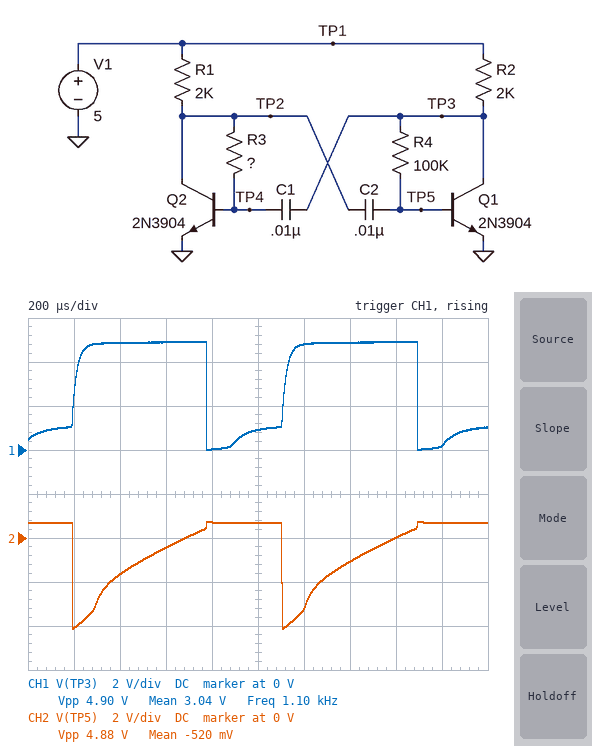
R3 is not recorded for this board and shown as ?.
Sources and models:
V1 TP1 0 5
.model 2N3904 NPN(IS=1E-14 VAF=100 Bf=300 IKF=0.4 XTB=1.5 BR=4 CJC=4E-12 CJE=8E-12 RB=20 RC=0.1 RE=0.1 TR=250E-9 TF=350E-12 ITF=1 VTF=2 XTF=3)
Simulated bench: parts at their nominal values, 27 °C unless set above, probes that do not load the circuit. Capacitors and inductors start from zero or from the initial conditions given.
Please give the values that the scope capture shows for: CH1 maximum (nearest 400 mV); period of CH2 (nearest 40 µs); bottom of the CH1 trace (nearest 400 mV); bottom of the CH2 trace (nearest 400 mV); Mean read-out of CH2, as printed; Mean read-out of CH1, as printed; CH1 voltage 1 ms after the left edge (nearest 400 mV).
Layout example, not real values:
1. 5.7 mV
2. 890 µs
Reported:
1. 4.8 V
2. 920 µs
3. 0 V
4. -4.0 V
5. -520 mV
6. 3.04 V
7. 800 mV
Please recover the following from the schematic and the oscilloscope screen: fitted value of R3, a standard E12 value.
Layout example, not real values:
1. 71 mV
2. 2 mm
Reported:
1. 56 kΩ
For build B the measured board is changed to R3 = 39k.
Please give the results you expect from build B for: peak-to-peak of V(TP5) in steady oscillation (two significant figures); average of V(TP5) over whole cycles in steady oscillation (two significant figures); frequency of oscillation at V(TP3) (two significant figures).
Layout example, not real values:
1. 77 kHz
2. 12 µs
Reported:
1. 4.8 V
2. -750 mV
3. 1.2 kHz
